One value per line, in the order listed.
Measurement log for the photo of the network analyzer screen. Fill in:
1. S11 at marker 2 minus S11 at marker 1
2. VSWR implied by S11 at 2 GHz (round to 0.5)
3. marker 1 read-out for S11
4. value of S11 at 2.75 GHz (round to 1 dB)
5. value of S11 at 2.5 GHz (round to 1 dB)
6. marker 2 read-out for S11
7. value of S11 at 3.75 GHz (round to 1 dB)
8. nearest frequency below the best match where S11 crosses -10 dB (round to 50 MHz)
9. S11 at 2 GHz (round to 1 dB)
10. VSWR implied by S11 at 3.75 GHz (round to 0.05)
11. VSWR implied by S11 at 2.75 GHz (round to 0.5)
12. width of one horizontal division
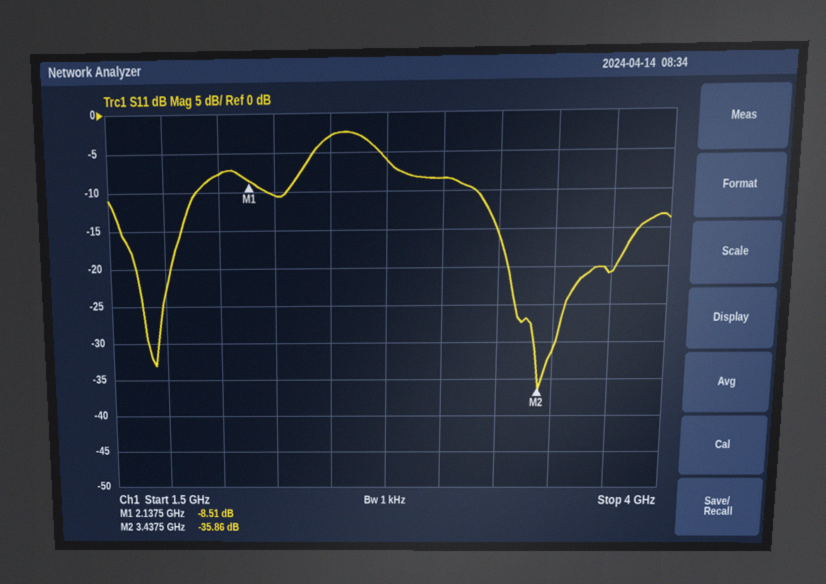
-27.35 dB
2.5
-8.51 dB
-6 dB
-3 dB
-35.86 dB
-21 dB
3.15 GHz
-8 dB
1.20
3.0
250 MHz
